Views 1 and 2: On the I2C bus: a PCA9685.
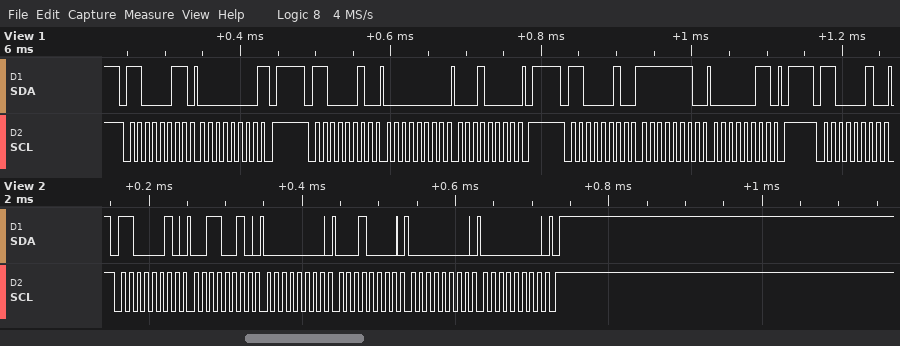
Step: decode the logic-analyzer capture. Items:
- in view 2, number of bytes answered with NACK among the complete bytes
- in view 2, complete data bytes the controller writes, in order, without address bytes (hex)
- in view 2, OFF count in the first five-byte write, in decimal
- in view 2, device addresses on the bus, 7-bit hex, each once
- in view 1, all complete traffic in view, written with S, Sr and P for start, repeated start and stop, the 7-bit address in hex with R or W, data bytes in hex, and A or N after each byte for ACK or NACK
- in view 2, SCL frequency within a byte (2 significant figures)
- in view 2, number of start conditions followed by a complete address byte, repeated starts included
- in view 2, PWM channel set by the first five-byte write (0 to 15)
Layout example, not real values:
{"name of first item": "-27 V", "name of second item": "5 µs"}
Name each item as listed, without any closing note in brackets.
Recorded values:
{"in view 2, number of bytes answered with NACK among the complete bytes": "0", "in view 2, complete data bytes the controller writes, in order, without address bytes": "32 00 10 00 00", "in view 2, OFF count in the first five-byte write, in decimal": "0", "in view 2, device addresses on the bus, 7-bit hex, each once": "0x61", "in view 1, all complete traffic in view, written with S, Sr and P for start, repeated start and stop, the 7-bit address in hex with R or W, data bytes in hex, and A or N after each byte for ACK or NACK": "S 61R A 00 N P S 61W A 00 A 10 A P S 61W A FE A 03 A P S 61W A", "in view 2, SCL frequency within a byte": "100 kHz", "in view 2, number of start conditions followed by a complete address byte, repeated starts included": "1", "in view 2, PWM channel set by the first five-byte write": "11"}
